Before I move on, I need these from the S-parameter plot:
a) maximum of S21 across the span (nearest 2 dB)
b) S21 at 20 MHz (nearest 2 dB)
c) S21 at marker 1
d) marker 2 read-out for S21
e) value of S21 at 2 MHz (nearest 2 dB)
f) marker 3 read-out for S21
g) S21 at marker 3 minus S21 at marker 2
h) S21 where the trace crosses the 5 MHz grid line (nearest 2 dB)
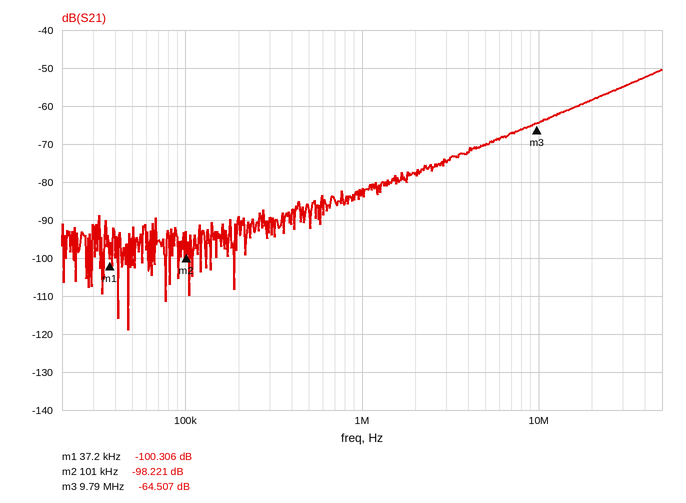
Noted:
-50 dB
-58 dB
-100.306 dB
-98.221 dB
-78 dB
-64.507 dB
33.714 dB
-70 dB
